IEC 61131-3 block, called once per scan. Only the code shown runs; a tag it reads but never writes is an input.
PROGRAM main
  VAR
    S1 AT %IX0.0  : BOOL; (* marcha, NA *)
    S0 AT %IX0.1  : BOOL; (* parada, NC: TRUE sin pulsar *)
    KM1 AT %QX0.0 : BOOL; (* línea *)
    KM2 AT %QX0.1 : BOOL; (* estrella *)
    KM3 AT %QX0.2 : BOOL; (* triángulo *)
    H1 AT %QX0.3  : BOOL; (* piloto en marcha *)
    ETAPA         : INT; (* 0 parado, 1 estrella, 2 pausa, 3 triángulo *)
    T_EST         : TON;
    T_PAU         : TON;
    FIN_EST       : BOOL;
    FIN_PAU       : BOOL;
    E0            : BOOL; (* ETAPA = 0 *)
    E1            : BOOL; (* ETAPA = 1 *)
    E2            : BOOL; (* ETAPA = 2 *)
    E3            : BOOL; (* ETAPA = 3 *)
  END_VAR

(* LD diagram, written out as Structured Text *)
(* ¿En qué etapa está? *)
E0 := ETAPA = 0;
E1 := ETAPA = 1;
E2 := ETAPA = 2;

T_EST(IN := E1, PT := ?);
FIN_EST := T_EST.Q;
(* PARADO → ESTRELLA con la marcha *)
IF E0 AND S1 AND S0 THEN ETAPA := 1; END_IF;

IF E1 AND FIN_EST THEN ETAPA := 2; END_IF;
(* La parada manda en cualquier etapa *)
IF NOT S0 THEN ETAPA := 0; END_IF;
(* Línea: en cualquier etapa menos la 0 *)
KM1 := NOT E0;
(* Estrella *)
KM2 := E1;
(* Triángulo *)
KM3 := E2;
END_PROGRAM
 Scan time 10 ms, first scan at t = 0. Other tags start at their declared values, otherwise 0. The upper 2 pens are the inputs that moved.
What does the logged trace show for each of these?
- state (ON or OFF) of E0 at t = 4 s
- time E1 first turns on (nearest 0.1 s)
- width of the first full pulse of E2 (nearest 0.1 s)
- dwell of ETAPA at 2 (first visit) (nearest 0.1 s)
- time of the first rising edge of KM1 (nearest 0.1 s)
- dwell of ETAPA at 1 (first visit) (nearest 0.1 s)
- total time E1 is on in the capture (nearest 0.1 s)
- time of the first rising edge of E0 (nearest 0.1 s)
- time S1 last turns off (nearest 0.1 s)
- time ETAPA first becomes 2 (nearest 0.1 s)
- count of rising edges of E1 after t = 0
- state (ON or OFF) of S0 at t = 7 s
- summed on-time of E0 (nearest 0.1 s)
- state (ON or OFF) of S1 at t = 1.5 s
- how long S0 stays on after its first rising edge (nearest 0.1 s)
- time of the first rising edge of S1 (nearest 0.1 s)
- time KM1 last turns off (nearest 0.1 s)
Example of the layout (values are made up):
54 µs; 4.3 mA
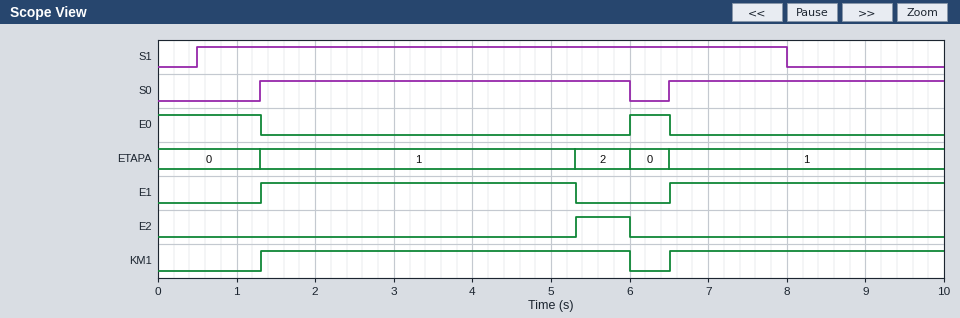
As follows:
OFF; 1.3 s; 0.7 s; 0.7 s; 1.3 s; 4.0 s; 7.5 s; 6.0 s; 8.0 s; 5.3 s; 2; ON; 1.8 s; ON; 4.7 s; 0.5 s; 6.0 s
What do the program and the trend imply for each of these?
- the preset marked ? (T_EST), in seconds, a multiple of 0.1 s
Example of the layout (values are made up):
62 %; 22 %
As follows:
4.0 s
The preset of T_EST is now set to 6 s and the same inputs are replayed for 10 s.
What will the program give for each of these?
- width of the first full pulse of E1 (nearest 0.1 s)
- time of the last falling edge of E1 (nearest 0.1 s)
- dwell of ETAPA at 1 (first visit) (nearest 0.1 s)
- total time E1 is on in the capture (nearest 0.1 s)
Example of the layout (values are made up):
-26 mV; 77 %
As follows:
4.7 s; 6.0 s; 4.7 s; 8.2 s
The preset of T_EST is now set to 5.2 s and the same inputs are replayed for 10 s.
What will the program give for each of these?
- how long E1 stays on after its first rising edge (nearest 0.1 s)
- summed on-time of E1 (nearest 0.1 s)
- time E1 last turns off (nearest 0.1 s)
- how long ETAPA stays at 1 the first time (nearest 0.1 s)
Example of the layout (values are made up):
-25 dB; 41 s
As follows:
4.7 s; 8.2 s; 6.0 s; 4.7 s
